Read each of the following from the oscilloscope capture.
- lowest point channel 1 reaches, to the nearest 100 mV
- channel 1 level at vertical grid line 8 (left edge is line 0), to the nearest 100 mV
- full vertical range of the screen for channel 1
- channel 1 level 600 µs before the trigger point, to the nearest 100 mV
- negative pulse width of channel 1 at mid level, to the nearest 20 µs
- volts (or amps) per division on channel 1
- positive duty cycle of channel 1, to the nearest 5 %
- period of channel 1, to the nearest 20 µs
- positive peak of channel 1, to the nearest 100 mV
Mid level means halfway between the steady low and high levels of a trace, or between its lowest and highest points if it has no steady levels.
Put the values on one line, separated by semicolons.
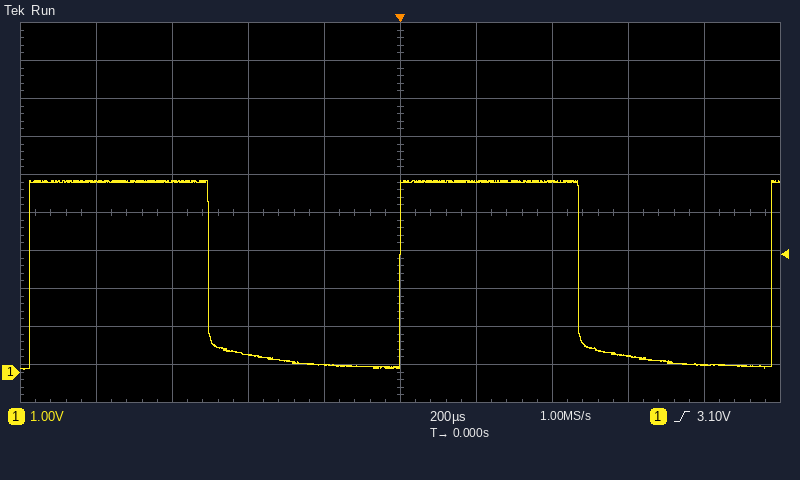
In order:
100 mV; 400 mV; 10 V; 5.0 V; 500 µs; 1 V; 50 %; 980 µs; 5.0 V
